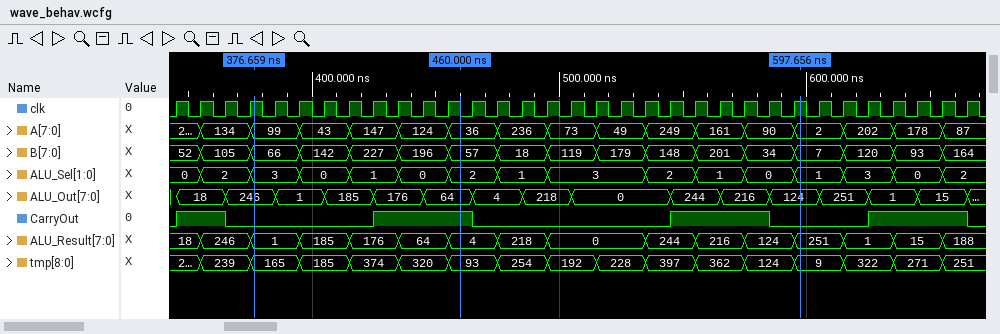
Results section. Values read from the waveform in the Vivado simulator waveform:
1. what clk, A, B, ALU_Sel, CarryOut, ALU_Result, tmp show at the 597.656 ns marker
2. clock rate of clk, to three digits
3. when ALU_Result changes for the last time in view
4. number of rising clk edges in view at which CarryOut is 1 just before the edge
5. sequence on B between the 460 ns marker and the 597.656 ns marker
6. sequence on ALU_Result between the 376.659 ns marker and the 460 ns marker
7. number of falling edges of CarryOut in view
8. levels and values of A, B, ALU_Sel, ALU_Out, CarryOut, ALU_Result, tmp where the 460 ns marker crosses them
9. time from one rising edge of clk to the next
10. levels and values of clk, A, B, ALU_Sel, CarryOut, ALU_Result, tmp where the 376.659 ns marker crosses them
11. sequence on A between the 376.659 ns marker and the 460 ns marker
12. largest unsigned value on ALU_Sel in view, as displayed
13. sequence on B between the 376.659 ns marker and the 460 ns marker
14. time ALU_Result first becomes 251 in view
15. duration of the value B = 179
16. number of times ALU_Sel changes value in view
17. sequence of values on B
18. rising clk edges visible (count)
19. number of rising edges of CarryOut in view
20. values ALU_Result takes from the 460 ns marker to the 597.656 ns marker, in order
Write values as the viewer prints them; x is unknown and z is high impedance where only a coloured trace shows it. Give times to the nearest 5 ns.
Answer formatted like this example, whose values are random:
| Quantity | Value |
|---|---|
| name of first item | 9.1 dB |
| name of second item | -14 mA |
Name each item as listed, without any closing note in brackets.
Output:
| Quantity | Value |
|---|---|
| what clk, A, B, ALU_Sel, CarryOut, ALU_Result, tmp show at the 597.656 ns marker | clk=1, A=2, B=7, ALU_Sel=1, CarryOut=0, ALU_Result=251, tmp=9 |
| clock rate of clk, to three digits | 100 MHz |
| when ALU_Result changes for the last time in view | 655 ns |
| number of rising clk edges in view at which CarryOut is 1 just before the edge | 14 |
| sequence on B between the 460 ns marker and the 597.656 ns marker | 57, 18, 119, 179, 148, 201, 34, 7 |
| sequence on ALU_Result between the 376.659 ns marker and the 460 ns marker | 1, 185, 176, 64, 4 |
| number of falling edges of CarryOut in view | 4 |
| levels and values of A, B, ALU_Sel, ALU_Out, CarryOut, ALU_Result, tmp where the 460 ns marker crosses them | A=36, B=57, ALU_Sel=2, ALU_Out=64, CarryOut=1, ALU_Result=4, tmp=93 |
| time from one rising edge of clk to the next | 10 ns |
| levels and values of clk, A, B, ALU_Sel, CarryOut, ALU_Result, tmp where the 376.659 ns marker crosses them | clk=1, A=99, B=66, ALU_Sel=3, CarryOut=0, ALU_Result=1, tmp=165 |
| sequence on A between the 376.659 ns marker and the 460 ns marker | 99, 43, 147, 124, 36 |
| largest unsigned value on ALU_Sel in view, as displayed | 3 |
| sequence on B between the 376.659 ns marker and the 460 ns marker | 66, 142, 227, 196, 57 |
| time ALU_Result first becomes 251 in view | 595 ns |
| duration of the value B = 179 | 20 ns |
| number of times ALU_Sel changes value in view | 15 |
| sequence of values on B | 52, 105, 66, 142, 227, 196, 57, 18, 119, 179, 148, 201, 34, 7, 120, 93, 164 |
| rising clk edges visible | 33 |
| number of rising edges of CarryOut in view | 4 |
| values ALU_Result takes from the 460 ns marker to the 597.656 ns marker, in order | 4, 218, 0, 244, 216, 124, 251 |
